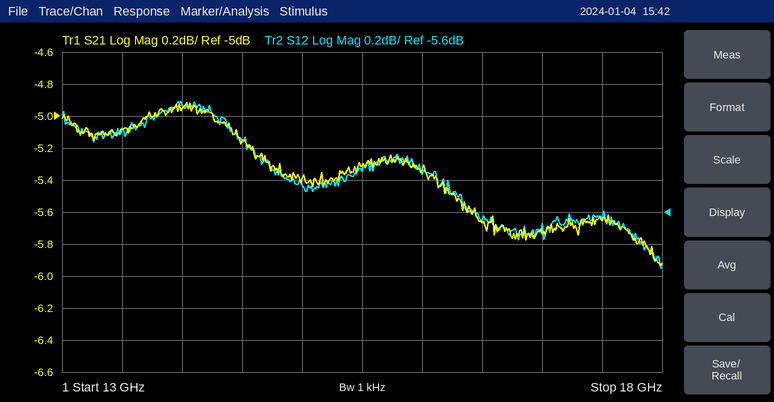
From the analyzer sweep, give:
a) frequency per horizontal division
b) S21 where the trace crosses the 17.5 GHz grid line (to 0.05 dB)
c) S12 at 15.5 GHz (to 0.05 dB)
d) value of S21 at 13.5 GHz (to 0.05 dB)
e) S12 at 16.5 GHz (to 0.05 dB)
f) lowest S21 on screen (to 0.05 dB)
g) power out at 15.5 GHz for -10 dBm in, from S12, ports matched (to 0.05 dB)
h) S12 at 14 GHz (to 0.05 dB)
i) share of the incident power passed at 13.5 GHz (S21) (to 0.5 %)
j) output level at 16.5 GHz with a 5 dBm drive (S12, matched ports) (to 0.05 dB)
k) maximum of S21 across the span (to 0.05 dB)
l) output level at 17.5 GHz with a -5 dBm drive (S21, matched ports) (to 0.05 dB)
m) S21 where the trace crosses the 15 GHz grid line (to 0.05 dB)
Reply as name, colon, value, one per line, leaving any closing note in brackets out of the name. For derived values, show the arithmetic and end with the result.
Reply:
frequency per horizontal division: 500 MHz
S21 where the trace crosses the 17.5 GHz grid line: -5.65 dB
S12 at 15.5 GHz: -5.35 dB
value of S21 at 13.5 GHz: -5.10 dB
S12 at 16.5 GHz: -5.65 dB
lowest S21 on screen: -5.95 dB
power out at 15.5 GHz for -10 dBm in, from S12, ports matched: -10 dBm + (-5.35 dB) = -15.35 dBm
S12 at 14 GHz: -4.95 dB
share of the incident power passed at 13.5 GHz (S21): 10^(-5.1/10) ≈ 30.9 %, so 31.0 % to the nearest 0.5 %
output level at 16.5 GHz with a 5 dBm drive (S12, matched ports): 5 dBm + (-5.65 dB) = -0.65 dBm
maximum of S21 across the span: -4.90 dB
output level at 17.5 GHz with a -5 dBm drive (S21, matched ports): -5 dBm + (-5.65 dB) = -10.65 dBm
S21 where the trace crosses the 15 GHz grid line: -5.40 dB
